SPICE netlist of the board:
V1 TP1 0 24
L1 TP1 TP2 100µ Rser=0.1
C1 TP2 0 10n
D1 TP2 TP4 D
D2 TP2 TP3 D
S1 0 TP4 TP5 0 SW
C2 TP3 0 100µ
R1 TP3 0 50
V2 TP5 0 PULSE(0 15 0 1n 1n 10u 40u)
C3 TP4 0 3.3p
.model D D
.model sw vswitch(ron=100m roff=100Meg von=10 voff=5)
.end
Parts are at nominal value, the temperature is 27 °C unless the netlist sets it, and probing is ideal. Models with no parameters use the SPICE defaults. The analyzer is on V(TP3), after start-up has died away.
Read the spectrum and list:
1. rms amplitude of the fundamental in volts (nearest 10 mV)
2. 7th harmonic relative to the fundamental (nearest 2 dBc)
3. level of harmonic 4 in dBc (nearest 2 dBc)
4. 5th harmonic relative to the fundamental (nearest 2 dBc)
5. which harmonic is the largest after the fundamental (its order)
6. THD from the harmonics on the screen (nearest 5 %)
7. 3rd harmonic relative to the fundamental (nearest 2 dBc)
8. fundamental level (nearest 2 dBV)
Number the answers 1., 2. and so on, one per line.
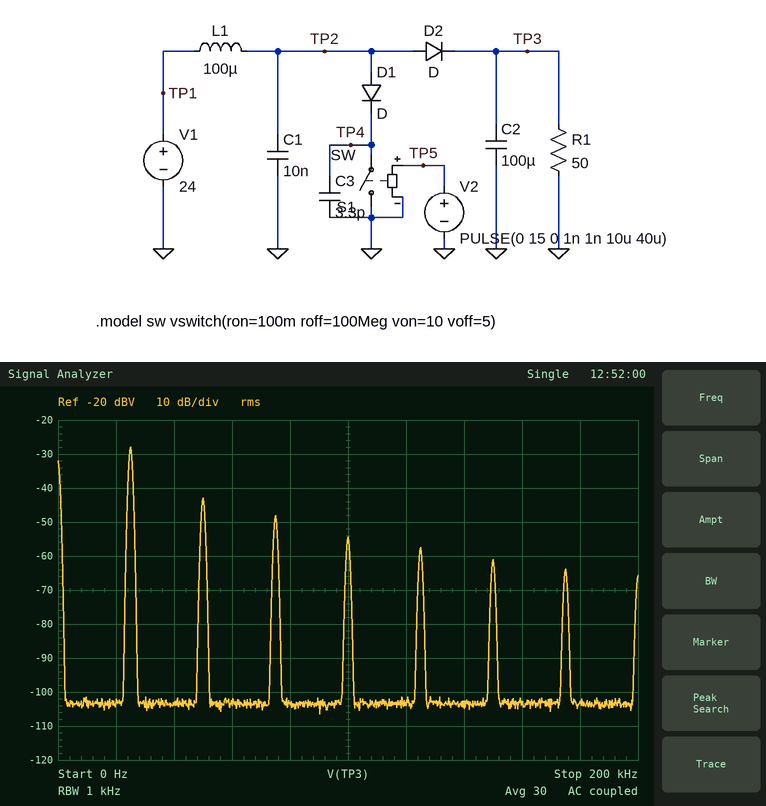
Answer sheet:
1. 40 mV
2. -36 dBc
3. -26 dBc
4. -30 dBc
5. 2
6. 20 %
7. -20 dBc
8. -28 dBV
